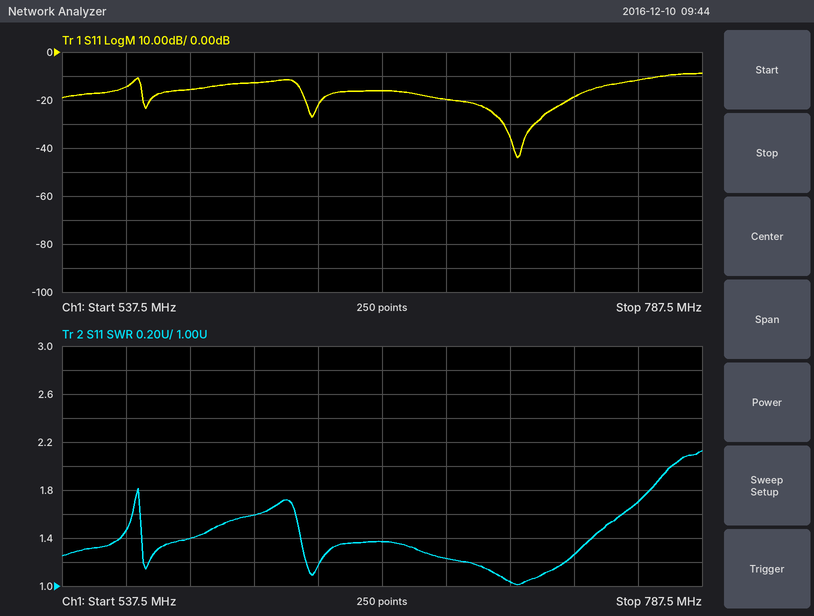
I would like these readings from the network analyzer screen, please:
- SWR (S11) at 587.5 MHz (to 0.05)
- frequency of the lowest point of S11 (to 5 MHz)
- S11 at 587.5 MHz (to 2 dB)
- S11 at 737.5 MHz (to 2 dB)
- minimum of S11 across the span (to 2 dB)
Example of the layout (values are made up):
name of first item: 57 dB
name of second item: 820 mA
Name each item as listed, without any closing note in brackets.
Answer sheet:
SWR (S11) at 587.5 MHz: 1.40
frequency of the lowest point of S11: 715 MHz
S11 at 587.5 MHz: -16 dB
S11 at 737.5 MHz: -18 dB
minimum of S11 across the span: -44 dB
